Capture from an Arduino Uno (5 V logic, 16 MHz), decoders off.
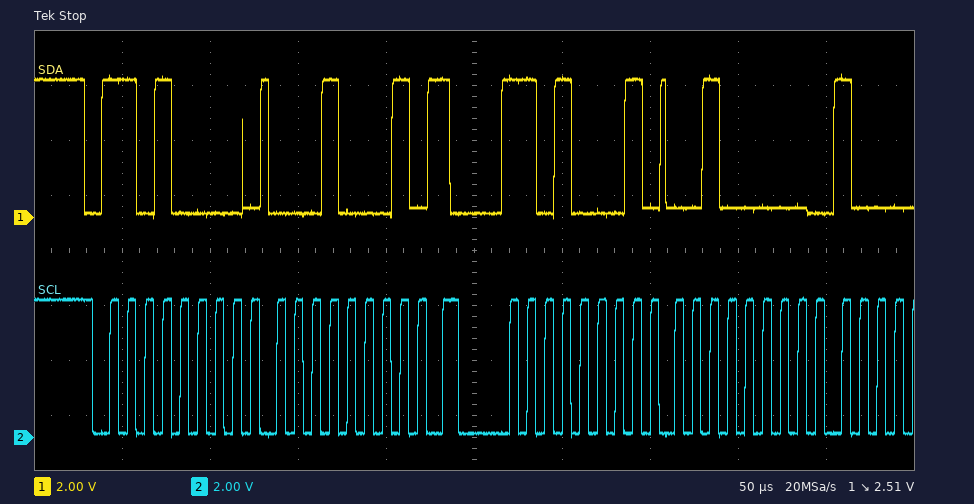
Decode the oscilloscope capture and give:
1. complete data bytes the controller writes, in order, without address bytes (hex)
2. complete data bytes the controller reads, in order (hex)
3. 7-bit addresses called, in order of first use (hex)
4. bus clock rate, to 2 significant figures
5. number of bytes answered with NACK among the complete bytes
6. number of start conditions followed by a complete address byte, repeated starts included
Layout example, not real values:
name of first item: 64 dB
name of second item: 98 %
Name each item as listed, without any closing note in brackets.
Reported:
complete data bytes the controller writes, in order, without address bytes: 11
complete data bytes the controller reads, in order: 20
7-bit addresses called, in order of first use: 0x68
bus clock rate, to 2 significant figures: 100 kHz
number of bytes answered with NACK among the complete bytes: 0
number of start conditions followed by a complete address byte, repeated starts included: 2
